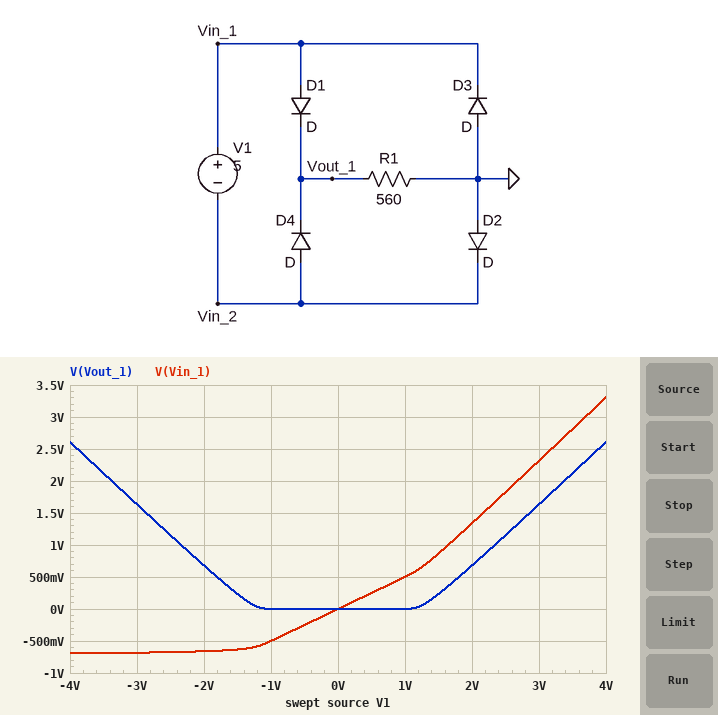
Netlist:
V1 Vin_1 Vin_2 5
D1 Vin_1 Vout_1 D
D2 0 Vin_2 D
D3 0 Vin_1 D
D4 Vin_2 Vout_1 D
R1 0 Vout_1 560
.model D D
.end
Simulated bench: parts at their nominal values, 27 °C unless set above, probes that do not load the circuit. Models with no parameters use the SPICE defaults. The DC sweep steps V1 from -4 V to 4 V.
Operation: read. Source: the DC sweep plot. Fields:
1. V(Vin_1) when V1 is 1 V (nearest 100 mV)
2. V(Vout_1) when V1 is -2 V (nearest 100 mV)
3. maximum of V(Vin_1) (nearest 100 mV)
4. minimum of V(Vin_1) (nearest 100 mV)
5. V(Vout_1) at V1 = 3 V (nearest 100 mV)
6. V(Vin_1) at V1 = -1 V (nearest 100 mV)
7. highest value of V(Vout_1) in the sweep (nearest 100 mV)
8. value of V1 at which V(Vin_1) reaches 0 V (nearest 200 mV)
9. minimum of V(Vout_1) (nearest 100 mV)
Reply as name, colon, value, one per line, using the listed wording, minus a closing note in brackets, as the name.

V(Vin_1) when V1 is 1 V: 500 mV
V(Vout_1) when V1 is -2 V: 700 mV
maximum of V(Vin_1): 3.3 V
minimum of V(Vin_1): -700 mV
V(Vout_1) at V1 = 3 V: 1.6 V
V(Vin_1) at V1 = -1 V: -500 mV
highest value of V(Vout_1) in the sweep: 2.6 V
value of V1 at which V(Vin_1) reaches 0 V: 0 V
minimum of V(Vout_1): 0 V
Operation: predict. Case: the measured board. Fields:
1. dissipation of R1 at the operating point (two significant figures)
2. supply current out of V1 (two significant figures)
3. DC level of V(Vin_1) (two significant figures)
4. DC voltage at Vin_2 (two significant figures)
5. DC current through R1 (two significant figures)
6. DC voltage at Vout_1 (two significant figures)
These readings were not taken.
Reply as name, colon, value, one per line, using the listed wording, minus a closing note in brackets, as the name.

dissipation of R1 at the operating point: 23 mW
supply current out of V1: 6.4 mA
DC level of V(Vin_1): 4.3 V
DC voltage at Vin_2: -700 mV
DC current through R1: 6.4 mA
DC voltage at Vout_1: 3.6 V
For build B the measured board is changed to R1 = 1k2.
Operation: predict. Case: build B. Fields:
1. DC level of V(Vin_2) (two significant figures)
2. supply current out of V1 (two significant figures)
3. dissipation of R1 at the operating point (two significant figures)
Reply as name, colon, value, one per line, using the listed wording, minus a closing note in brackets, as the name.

DC level of V(Vin_2): -680 mV
supply current out of V1: 3.0 mA
dissipation of R1 at the operating point: 11 mW
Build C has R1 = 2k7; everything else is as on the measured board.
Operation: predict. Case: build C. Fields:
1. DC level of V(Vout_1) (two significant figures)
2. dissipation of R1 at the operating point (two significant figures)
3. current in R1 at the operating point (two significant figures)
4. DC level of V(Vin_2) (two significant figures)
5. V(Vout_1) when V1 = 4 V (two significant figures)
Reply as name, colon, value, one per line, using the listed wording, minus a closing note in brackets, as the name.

DC level of V(Vout_1): 3.7 V
dissipation of R1 at the operating point: 5.0 mW
current in R1 at the operating point: 1.4 mA
DC level of V(Vin_2): -660 mV
V(Vout_1) when V1 = 4 V: 2.7 V
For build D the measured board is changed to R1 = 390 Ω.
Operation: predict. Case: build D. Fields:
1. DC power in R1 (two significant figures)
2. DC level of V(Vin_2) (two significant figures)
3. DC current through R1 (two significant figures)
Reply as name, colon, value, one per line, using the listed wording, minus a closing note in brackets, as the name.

DC power in R1: 33 mW
DC level of V(Vin_2): -710 mV
DC current through R1: 9.2 mA
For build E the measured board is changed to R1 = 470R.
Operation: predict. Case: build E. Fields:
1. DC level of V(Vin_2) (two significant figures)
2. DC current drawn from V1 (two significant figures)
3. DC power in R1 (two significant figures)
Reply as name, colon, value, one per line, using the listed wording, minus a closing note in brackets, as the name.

DC level of V(Vin_2): -710 mV
DC current drawn from V1: 7.6 mA
DC power in R1: 27 mW
